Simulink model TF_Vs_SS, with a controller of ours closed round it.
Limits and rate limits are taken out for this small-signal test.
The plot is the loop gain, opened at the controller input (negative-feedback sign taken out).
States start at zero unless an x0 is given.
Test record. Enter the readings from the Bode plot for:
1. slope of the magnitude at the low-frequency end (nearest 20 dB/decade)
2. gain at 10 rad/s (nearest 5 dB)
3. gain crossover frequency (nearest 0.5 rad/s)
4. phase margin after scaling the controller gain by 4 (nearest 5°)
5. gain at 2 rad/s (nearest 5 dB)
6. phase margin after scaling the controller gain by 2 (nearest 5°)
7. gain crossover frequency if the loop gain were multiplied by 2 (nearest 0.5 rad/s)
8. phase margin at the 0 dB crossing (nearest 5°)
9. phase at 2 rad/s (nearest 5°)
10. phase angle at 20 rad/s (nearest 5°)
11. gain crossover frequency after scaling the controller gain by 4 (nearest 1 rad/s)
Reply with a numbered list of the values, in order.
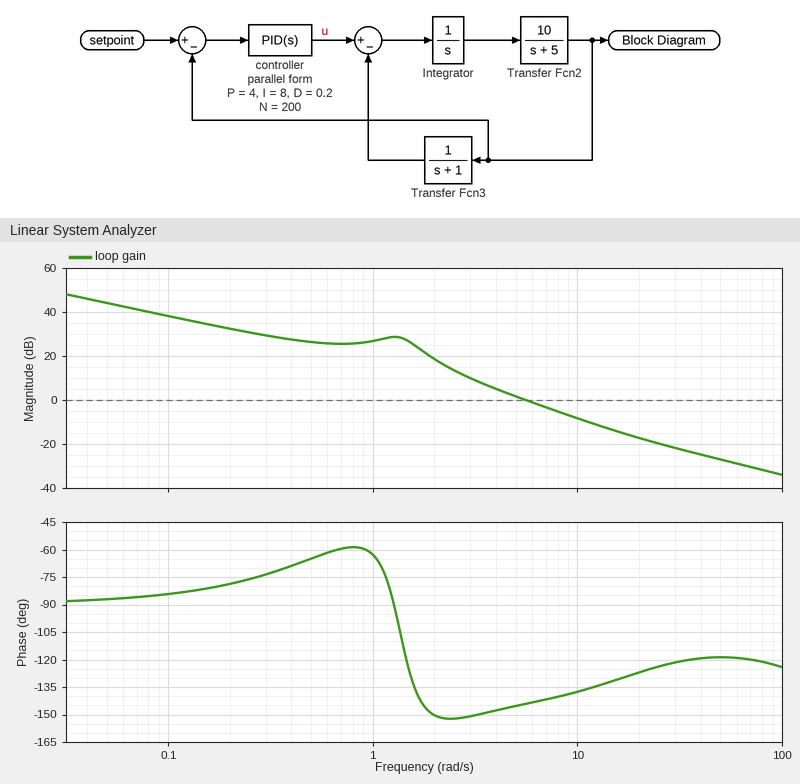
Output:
1. -20 dB/decade
2. -10 dB
3. 5.5 rad/s
4. 45°
5. 20 dB
6. 40°
7. 8.5 rad/s
8. 35°
9. -150°
10. -125°
11. 13 rad/s
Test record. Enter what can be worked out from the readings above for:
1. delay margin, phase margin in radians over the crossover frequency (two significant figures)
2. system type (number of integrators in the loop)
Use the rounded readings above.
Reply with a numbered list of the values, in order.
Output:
1. 0.11 s
2. 1
